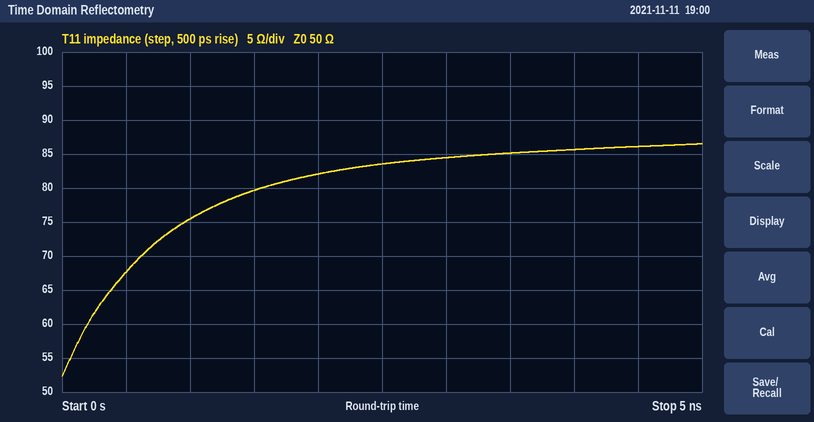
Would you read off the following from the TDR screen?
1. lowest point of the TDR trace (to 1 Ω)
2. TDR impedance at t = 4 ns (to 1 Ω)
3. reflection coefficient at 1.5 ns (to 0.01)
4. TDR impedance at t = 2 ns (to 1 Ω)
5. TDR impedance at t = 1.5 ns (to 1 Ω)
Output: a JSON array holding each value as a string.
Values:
["52 Ω", "86 Ω", "+0.23", "82 Ω", "80 Ω"]
